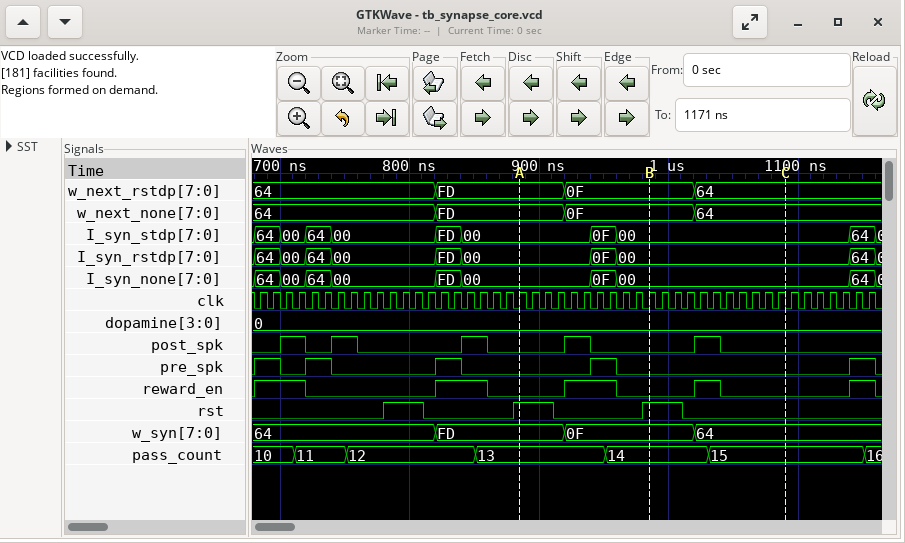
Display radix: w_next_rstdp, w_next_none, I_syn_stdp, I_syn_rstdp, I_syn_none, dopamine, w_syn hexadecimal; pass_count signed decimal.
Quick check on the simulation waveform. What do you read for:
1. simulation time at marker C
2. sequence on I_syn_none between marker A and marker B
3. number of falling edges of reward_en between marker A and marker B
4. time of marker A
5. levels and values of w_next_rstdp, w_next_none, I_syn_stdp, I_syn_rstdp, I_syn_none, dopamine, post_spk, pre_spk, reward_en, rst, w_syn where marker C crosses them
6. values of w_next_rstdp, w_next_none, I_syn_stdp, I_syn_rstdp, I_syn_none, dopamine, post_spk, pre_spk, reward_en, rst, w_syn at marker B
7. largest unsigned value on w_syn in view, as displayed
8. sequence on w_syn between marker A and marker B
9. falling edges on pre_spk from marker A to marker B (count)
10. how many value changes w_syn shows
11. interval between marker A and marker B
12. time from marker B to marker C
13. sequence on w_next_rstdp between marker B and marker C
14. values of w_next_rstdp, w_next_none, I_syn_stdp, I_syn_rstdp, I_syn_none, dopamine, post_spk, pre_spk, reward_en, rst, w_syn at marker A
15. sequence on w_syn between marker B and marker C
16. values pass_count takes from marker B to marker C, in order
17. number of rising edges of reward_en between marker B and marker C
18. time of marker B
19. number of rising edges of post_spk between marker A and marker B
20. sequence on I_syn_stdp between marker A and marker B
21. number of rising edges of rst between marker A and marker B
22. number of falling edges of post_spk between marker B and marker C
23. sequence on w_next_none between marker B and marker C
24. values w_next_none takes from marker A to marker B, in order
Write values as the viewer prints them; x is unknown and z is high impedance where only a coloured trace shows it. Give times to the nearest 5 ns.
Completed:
1090 ns
00, 0F, 00
1
885 ns
w_next_rstdp=64, w_next_none=64, I_syn_stdp=00, I_syn_rstdp=00, I_syn_none=00, dopamine=0, post_spk=0, pre_spk=0, reward_en=0, rst=0, w_syn=64
w_next_rstdp=0F, w_next_none=0F, I_syn_stdp=00, I_syn_rstdp=00, I_syn_none=00, dopamine=0, post_spk=0, pre_spk=0, reward_en=0, rst=1, w_syn=0F
FD
FD, 0F
1
3
100 ns
105 ns
0F, 64
w_next_rstdp=FD, w_next_none=FD, I_syn_stdp=00, I_syn_rstdp=00, I_syn_none=00, dopamine=0, post_spk=0, pre_spk=0, reward_en=0, rst=1, w_syn=FD
0F, 64
14, 15
1
985 ns
1
00, 0F, 00
1
1
0F, 64
FD, 0F
